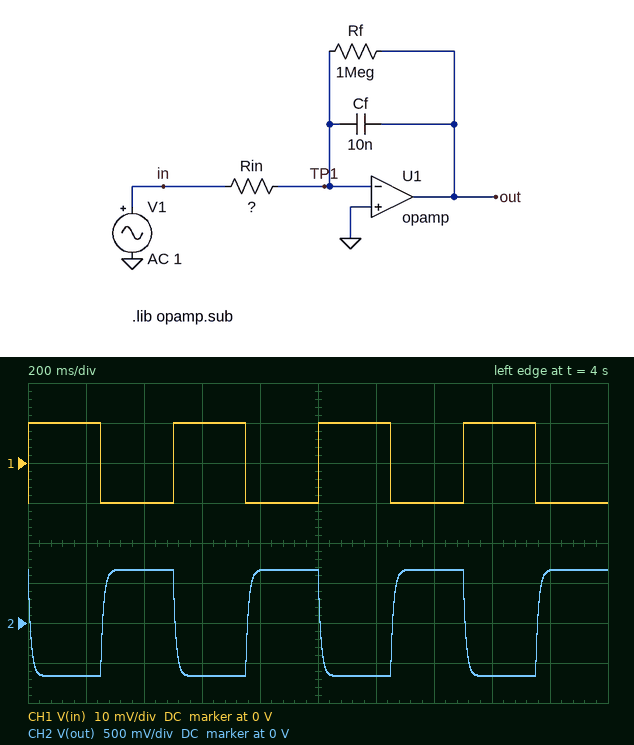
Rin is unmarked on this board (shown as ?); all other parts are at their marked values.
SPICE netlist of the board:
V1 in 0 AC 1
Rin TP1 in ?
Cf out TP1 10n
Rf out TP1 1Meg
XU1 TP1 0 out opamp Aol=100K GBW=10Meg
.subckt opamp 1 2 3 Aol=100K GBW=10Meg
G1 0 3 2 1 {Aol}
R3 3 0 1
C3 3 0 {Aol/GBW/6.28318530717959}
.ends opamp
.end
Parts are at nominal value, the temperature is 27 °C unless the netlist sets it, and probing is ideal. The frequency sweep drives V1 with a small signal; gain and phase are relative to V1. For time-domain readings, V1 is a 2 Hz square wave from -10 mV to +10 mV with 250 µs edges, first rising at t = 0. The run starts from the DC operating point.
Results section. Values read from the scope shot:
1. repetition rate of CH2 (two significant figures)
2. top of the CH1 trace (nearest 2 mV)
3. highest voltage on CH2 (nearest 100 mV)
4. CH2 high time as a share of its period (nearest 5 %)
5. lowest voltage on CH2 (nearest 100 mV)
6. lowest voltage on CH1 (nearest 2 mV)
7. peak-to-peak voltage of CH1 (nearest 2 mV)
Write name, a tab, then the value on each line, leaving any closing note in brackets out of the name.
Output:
repetition rate of CH2	2.0 Hz
top of the CH1 trace	10 mV
highest voltage on CH2	700 mV
CH2 high time as a share of its period	50 %
lowest voltage on CH2	-700 mV
lowest voltage on CH1	-10 mV
peak-to-peak voltage of CH1	20 mV
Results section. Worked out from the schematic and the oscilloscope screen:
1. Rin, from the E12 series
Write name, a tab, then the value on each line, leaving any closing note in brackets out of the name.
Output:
Rin, from the E12 series	15 kΩ
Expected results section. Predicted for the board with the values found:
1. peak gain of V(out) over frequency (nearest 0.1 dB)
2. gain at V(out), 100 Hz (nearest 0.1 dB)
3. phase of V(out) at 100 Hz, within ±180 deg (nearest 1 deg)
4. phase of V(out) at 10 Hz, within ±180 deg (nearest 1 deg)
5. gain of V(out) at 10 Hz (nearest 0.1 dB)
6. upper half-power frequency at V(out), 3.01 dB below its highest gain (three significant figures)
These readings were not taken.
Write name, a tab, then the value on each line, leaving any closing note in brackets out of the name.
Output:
peak gain of V(out) over frequency	36.5 dB
gain at V(out), 100 Hz	20.4 dB
phase of V(out) at 100 Hz, within ±180 deg	99 deg
phase of V(out) at 10 Hz, within ±180 deg	148 deg
gain of V(out) at 10 Hz	35.0 dB
upper half-power frequency at V(out), 3.01 dB below its highest gain	15.9 Hz
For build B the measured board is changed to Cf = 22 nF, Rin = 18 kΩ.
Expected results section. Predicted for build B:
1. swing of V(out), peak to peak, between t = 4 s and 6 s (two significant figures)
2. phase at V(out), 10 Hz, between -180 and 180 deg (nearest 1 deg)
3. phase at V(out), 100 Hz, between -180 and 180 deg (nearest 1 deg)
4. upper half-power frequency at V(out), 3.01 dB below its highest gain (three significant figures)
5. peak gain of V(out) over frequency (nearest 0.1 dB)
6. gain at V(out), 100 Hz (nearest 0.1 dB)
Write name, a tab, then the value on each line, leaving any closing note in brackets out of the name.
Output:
swing of V(out), peak to peak, between t = 4 s and 6 s	1.1 V
phase at V(out), 10 Hz, between -180 and 180 deg	126 deg
phase at V(out), 100 Hz, between -180 and 180 deg	94 deg
upper half-power frequency at V(out), 3.01 dB below its highest gain	7.24 Hz
peak gain of V(out) over frequency	34.9 dB
gain at V(out), 100 Hz	12.1 dB
